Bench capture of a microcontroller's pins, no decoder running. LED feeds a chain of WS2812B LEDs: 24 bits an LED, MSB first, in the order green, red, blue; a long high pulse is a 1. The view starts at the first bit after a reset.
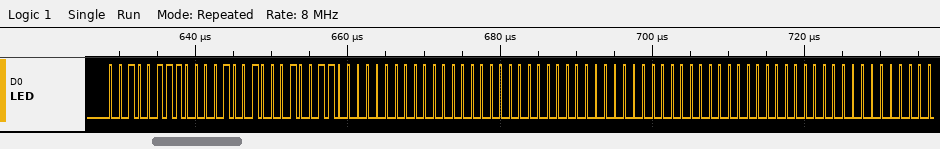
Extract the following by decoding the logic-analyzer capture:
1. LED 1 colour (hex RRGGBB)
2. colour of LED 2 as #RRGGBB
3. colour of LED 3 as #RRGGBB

#092713
#000000
#000000
